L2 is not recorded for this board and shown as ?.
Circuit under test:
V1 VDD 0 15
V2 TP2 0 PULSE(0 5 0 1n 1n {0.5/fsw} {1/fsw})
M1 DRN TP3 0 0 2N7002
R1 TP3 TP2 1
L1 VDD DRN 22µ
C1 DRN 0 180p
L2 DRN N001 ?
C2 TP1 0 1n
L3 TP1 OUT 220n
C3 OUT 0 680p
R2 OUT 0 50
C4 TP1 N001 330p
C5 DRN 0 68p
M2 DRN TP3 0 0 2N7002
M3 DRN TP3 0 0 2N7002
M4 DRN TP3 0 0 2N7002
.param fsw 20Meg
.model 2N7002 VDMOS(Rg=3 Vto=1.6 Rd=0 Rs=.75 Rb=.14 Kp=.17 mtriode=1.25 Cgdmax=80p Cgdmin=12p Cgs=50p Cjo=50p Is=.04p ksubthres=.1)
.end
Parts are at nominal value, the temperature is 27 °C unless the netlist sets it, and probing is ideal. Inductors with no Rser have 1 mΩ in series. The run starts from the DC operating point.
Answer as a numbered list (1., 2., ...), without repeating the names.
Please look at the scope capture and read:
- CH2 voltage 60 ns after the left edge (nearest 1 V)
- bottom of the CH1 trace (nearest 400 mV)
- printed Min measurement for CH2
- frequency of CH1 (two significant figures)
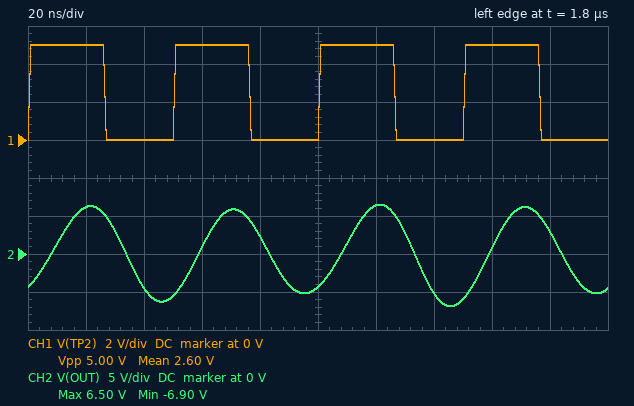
1. 1 V
2. 0 V
3. -6.90 V
4. 20 MHz
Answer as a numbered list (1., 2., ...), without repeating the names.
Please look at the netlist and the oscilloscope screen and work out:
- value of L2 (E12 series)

1. 150 nH
